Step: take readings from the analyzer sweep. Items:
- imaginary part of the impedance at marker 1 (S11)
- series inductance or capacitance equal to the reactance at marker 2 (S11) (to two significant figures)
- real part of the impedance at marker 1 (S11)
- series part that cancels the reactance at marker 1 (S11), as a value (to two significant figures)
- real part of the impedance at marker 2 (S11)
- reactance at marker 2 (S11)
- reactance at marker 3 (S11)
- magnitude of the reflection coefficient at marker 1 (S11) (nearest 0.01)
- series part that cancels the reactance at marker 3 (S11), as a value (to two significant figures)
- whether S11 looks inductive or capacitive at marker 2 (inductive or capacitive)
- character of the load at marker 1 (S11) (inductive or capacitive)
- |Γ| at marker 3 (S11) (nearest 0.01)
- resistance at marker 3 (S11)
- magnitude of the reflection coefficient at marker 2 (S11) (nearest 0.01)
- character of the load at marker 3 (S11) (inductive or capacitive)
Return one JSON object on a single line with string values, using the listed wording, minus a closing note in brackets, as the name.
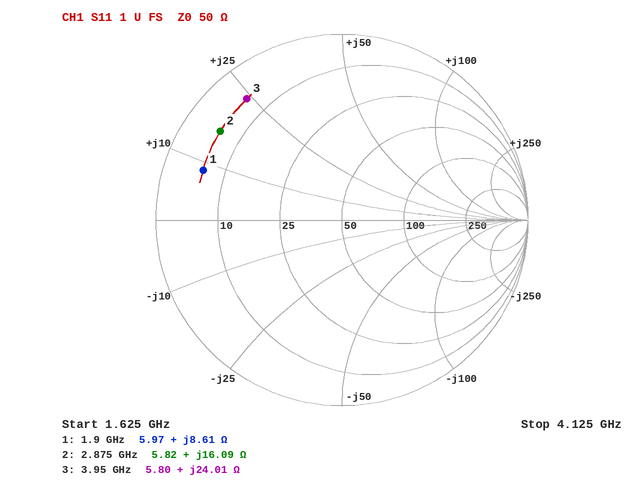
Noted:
{"imaginary part of the impedance at marker 1": "+8.61 Ω", "series inductance or capacitance equal to the reactance at marker 2 (S11)": "890 pH", "real part of the impedance at marker 1": "5.97 Ω", "series part that cancels the reactance at marker 1 (S11), as a value": "9.7 pF", "real part of the impedance at marker 2": "5.82 Ω", "reactance at marker 2": "+16.09 Ω", "reactance at marker 3": "+24.01 Ω", "magnitude of the reflection coefficient at marker 1 (S11)": "0.79", "series part that cancels the reactance at marker 3 (S11), as a value": "1.7 pF", "whether S11 looks inductive or capacitive at marker 2": "inductive", "character of the load at marker 1 (S11)": "inductive", "|Γ| at marker 3 (S11)": "0.83", "resistance at marker 3": "5.80 Ω", "magnitude of the reflection coefficient at marker 2 (S11)": "0.81", "character of the load at marker 3 (S11)": "inductive"}
